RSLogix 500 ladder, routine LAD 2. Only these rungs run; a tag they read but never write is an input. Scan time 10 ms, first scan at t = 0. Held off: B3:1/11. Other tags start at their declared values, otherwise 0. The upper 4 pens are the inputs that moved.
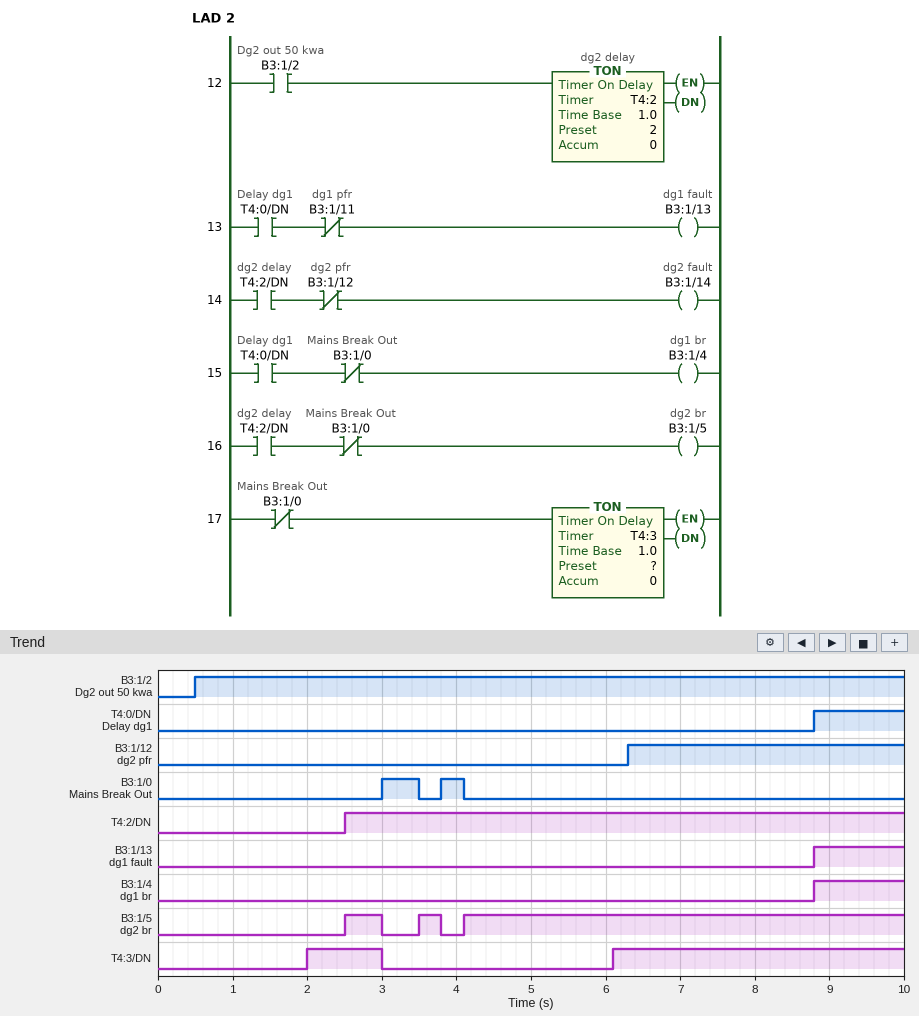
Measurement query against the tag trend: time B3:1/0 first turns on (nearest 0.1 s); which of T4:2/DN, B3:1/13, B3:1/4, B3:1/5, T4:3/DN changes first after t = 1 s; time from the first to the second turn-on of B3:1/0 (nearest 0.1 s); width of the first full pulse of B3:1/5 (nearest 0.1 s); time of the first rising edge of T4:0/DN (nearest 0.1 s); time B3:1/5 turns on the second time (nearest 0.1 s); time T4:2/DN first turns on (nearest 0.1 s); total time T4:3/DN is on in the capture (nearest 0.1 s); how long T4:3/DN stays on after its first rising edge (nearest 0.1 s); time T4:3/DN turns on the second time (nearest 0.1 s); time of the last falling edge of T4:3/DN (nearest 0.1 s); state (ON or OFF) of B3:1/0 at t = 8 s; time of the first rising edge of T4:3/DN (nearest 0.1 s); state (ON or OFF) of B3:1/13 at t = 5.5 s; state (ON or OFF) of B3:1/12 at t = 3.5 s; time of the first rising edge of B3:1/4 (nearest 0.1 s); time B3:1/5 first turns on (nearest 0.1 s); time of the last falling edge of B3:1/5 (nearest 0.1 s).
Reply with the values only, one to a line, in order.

3.0 s
T4:3/DN
0.8 s
0.5 s
8.8 s
3.5 s
2.5 s
4.9 s
1.0 s
6.1 s
3.0 s
OFF
2.0 s
OFF
OFF
8.8 s
2.5 s
3.8 s
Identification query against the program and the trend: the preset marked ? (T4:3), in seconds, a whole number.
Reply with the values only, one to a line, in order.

2 s
